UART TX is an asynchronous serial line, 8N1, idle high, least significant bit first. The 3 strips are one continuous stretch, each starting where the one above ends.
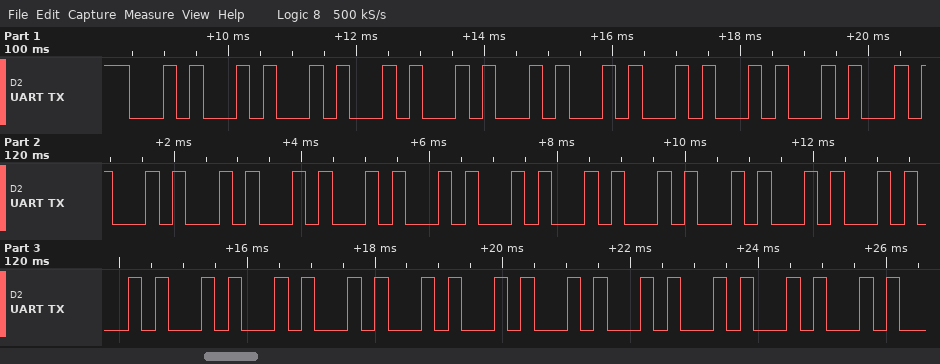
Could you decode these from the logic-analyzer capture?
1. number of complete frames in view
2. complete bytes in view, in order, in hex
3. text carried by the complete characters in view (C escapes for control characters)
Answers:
33
30 30 30 30 30 30 30 30 30 30 30 30 30 30 30 30 30 30 30 30 30 30 30 30 30 30 30 30 30 30 30 30 30
"000000000000000000000000000000000"
